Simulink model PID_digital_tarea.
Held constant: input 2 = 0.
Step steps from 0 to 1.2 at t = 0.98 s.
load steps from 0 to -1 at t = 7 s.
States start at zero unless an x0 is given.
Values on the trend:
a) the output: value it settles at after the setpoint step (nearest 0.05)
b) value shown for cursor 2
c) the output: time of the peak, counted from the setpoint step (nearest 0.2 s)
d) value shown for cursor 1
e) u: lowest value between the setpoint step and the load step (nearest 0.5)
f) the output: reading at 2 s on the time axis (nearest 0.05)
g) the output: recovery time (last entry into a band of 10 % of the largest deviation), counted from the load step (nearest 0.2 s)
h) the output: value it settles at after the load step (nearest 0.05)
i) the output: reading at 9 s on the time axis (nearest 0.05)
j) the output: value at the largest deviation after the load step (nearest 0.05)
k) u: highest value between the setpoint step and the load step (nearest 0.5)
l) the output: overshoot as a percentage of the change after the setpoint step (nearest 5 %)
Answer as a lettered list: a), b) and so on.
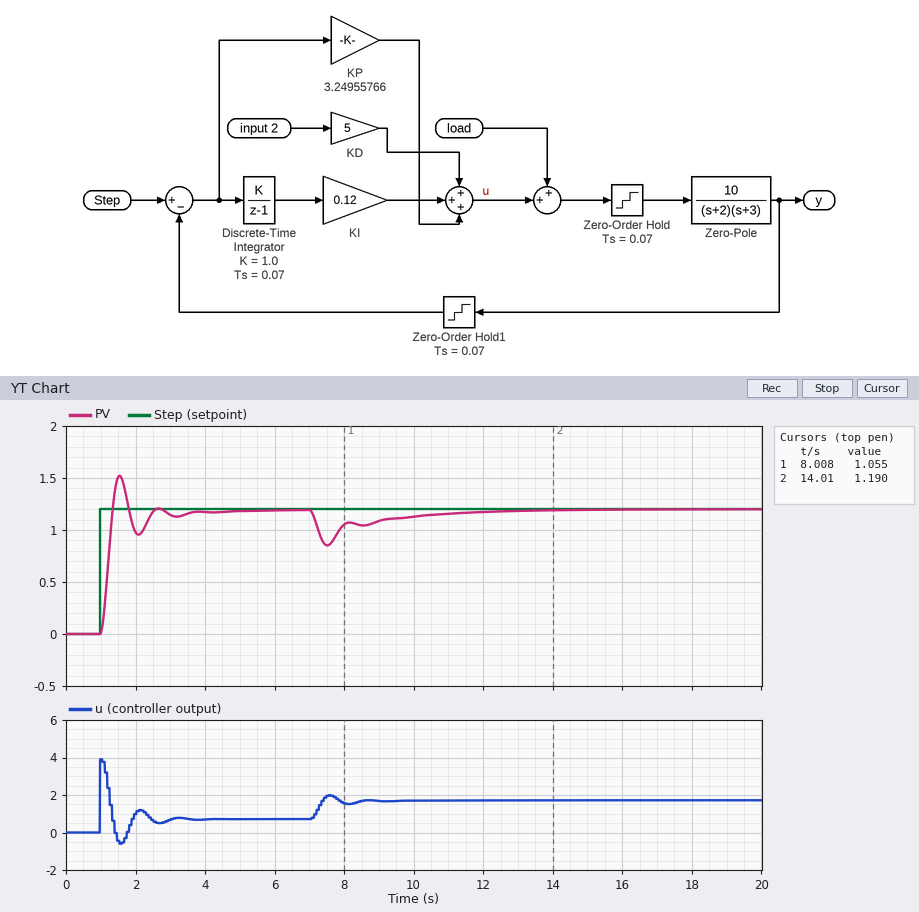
a) 1.20
b) 1.190
c) 0.6 s
d) 1.055
e) -0.5
f) 1.00
g) 4.6 s
h) 1.20
i) 1.10
j) 0.85
k) 4.0
l) 25 %
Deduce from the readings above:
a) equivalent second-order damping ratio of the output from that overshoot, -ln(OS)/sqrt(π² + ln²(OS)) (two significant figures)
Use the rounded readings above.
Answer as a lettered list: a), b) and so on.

a) 0.40
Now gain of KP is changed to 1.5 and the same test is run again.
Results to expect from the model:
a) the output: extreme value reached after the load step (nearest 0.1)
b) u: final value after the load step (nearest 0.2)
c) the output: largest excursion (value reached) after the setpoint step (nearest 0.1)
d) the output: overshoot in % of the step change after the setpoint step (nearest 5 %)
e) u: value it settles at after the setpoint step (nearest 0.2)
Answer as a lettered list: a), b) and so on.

a) 0.7
b) 1.8
c) 1.4
d) 15 %
e) 0.8
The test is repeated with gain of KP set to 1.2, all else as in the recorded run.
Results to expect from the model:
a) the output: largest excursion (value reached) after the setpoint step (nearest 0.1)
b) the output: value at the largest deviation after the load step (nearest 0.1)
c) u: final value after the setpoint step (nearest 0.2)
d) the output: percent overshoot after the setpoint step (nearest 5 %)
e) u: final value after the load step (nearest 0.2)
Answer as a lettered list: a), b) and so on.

a) 1.4
b) 0.6
c) 0.8
d) 15 %
e) 1.8
